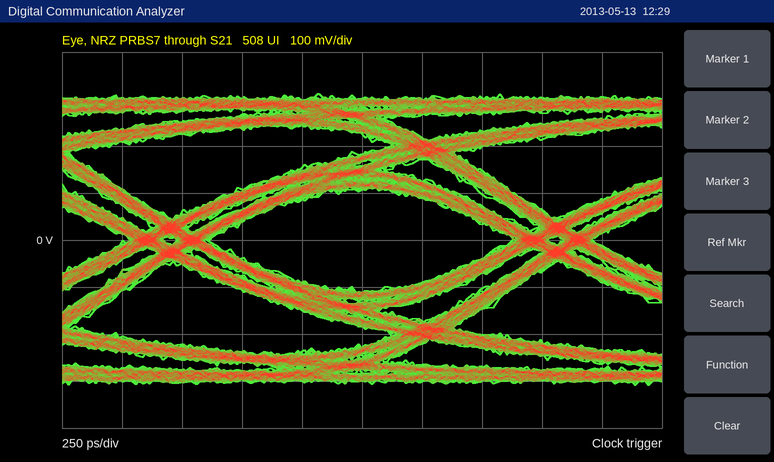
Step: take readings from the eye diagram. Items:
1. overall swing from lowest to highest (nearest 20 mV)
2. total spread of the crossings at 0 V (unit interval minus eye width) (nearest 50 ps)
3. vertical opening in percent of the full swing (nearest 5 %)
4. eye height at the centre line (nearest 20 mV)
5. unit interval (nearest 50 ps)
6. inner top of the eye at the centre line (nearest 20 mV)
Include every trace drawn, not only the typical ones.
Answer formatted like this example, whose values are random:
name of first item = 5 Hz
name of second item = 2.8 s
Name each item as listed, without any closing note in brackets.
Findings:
overall swing from lowest to highest = 620 mV
total spread of the crossings at 0 V (unit interval minus eye width) = 350 ps
vertical opening in percent of the full swing = 35 %
eye height at the centre line = 220 mV
unit interval = 1.60 ns
inner top of the eye at the centre line = 100 mV
